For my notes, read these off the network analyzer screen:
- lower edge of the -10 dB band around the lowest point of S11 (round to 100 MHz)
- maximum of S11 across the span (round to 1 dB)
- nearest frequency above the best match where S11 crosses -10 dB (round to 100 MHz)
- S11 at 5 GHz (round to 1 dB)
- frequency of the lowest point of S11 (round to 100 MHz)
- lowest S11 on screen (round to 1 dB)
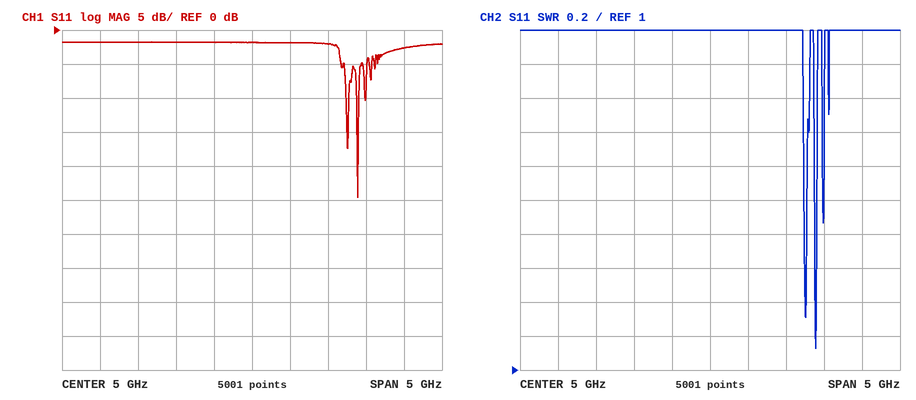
6.4 GHz
-2 dB
6.4 GHz
-2 dB
6.4 GHz
-25 dB
